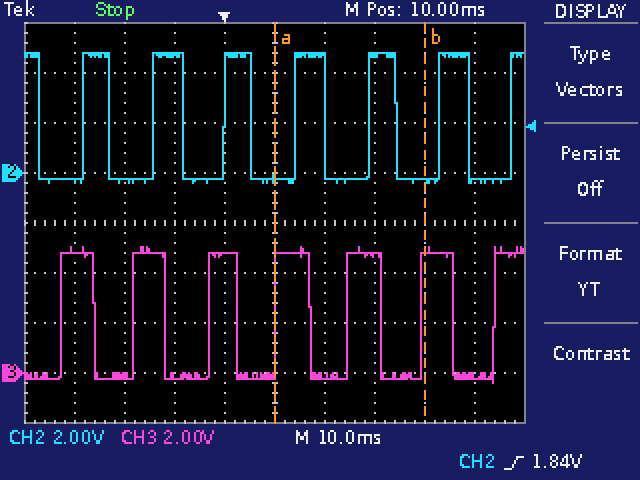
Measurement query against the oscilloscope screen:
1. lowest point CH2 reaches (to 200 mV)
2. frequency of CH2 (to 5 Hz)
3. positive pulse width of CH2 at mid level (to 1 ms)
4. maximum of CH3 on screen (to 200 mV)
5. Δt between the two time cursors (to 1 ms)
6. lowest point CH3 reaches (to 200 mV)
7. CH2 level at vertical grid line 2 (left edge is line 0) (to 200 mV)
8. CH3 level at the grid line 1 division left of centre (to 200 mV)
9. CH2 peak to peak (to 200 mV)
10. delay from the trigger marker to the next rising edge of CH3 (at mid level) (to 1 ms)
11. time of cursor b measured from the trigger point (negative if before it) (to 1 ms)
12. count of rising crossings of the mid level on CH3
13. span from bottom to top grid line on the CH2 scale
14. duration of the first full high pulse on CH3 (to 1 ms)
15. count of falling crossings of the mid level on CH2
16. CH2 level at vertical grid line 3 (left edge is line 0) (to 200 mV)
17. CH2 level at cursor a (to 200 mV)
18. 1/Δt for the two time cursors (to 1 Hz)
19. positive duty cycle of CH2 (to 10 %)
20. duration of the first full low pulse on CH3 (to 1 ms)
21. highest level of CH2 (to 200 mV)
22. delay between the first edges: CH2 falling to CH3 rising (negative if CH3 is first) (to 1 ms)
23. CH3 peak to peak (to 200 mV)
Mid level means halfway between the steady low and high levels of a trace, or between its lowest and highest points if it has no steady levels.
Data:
-400 mV
70 Hz
6 ms
5.0 V
30 ms
-400 mV
-200 mV
4.8 V
5.2 V
10 ms
+40 ms
7
16 V
7 ms
7
4.8 V
-200 mV
33 Hz
40 %
8 ms
4.8 V
+4 ms
5.4 V
